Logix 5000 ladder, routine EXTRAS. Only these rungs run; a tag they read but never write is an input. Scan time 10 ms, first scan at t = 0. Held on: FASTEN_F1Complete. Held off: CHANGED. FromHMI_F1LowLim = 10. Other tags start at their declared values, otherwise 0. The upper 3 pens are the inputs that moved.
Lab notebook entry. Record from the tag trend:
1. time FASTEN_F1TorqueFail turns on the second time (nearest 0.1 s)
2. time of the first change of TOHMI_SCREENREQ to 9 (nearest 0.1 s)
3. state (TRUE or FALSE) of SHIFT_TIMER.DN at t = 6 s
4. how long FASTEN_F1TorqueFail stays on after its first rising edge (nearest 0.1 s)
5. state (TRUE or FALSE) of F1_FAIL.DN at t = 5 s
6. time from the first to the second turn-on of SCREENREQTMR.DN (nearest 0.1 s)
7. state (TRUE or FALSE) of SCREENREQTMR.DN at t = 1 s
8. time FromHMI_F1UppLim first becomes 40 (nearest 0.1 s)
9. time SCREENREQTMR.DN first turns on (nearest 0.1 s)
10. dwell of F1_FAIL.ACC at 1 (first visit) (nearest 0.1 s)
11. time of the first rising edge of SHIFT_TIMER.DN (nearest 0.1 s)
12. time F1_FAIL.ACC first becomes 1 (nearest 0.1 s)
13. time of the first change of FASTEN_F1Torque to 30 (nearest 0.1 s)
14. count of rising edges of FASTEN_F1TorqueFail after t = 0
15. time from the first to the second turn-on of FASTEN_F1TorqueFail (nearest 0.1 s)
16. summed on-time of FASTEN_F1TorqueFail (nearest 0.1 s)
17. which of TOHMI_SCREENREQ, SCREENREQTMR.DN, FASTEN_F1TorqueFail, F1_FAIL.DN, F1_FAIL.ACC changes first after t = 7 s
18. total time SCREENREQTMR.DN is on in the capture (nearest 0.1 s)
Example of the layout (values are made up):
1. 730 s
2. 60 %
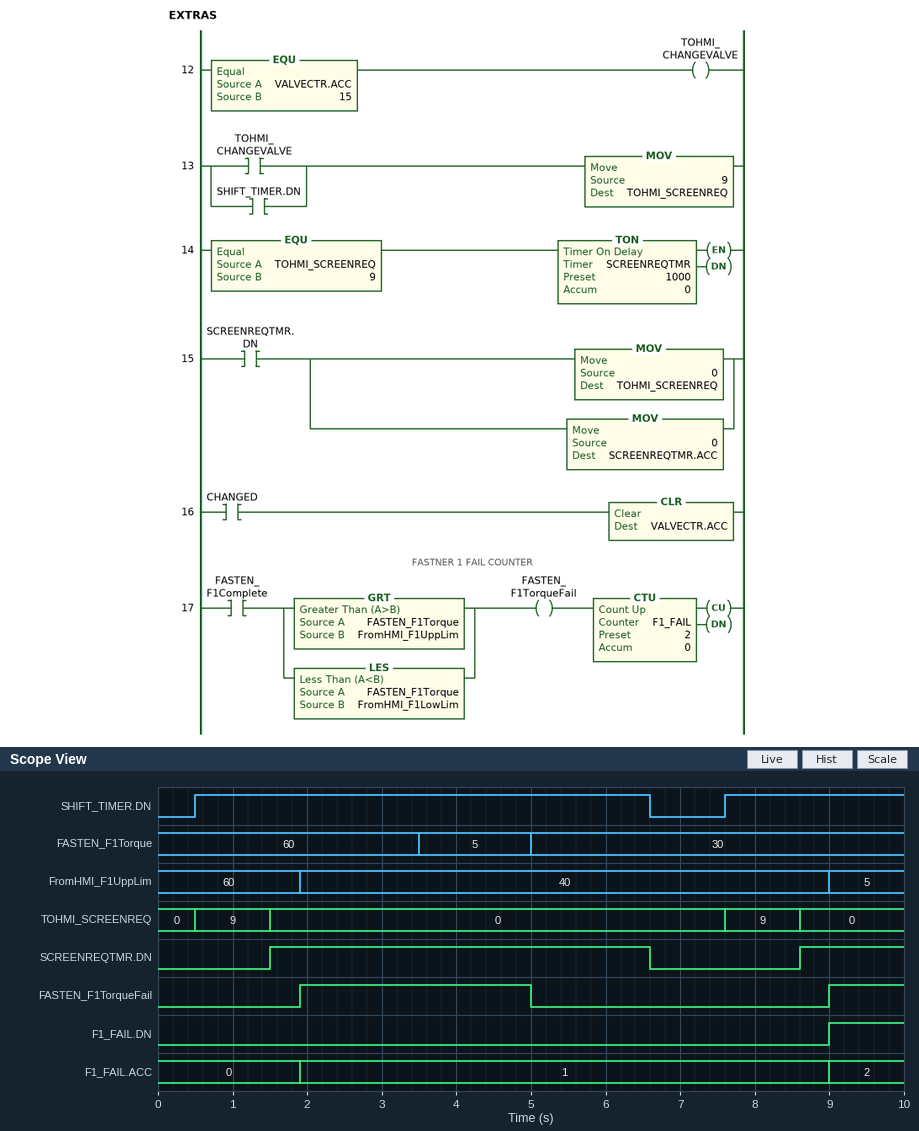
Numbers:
1. 9.0 s
2. 0.5 s
3. TRUE
4. 3.1 s
5. FALSE
6. 7.1 s
7. FALSE
8. 1.9 s
9. 1.5 s
10. 7.1 s
11. 0.5 s
12. 1.9 s
13. 5.0 s
14. 2
15. 7.1 s
16. 4.1 s
17. TOHMI_SCREENREQ
18. 6.5 s
